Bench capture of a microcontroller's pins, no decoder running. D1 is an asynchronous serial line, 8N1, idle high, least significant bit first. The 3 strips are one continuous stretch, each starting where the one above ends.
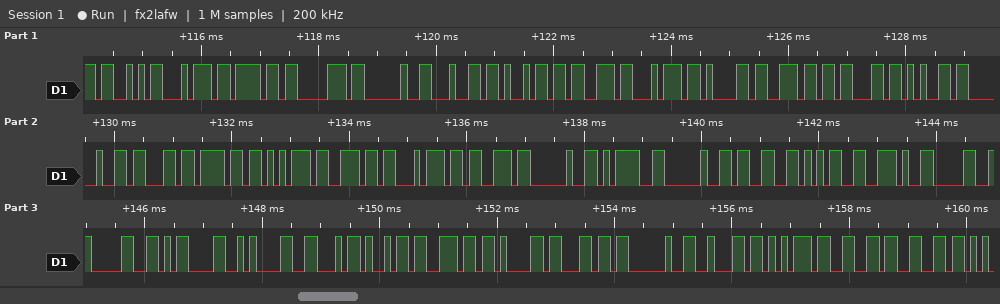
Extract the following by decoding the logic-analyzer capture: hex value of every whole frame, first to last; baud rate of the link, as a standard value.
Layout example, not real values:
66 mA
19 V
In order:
53 74 6F 70 20 64 69 73 74 61 6E 63 65 20 63 6F 75 6E 74 73 20 3D 20 33 35 2E 30 30 0D 0A 46 69 6E 61 6C 20 62 75 66 66
9600 baud
